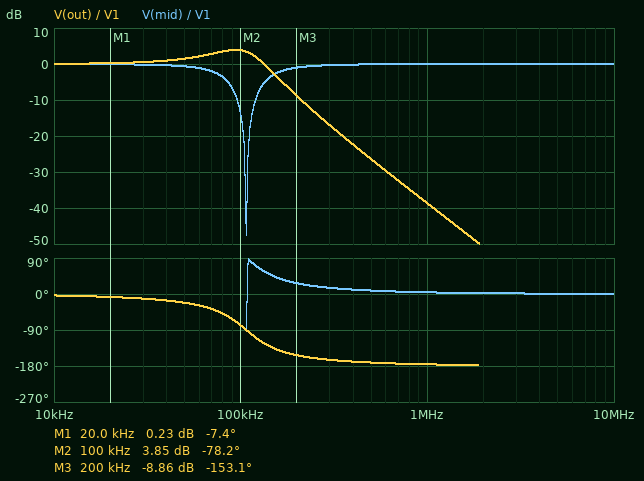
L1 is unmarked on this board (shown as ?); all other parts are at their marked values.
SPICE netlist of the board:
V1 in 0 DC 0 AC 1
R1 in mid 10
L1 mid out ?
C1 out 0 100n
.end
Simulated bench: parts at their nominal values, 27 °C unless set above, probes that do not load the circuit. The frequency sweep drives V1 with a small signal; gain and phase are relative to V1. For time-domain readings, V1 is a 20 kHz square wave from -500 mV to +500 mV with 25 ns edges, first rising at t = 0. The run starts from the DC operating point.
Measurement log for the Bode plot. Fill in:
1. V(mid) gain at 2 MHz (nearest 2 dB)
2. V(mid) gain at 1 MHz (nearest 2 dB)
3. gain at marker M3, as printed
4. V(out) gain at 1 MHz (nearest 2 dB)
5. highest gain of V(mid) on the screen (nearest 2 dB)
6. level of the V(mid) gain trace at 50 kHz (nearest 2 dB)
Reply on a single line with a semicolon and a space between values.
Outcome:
0 dB; 0 dB; -8.86 dB; -38 dB; 0 dB; 0 dB
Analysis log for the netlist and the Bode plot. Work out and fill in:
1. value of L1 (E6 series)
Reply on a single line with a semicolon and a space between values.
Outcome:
22 µH
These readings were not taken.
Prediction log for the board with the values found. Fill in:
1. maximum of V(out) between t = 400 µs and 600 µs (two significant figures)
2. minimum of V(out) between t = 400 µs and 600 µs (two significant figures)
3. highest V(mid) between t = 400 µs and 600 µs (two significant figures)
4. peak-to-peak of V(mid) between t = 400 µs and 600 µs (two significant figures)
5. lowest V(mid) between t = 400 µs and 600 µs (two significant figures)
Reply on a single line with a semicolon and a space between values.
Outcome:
830 mV; -830 mV; 640 mV; 1.3 V; -640 mV
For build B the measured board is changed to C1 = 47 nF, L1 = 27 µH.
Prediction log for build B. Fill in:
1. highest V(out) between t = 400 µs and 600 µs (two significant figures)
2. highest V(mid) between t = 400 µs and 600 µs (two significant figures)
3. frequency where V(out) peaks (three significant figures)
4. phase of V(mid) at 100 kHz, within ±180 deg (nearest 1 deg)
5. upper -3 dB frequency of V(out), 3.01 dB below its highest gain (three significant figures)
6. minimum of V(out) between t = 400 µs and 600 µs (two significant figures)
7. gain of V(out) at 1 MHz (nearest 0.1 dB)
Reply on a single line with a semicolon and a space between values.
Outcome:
1.0 V; 660 mV; 135 kHz; -31 deg; 162 kHz; -1.0 V; -33.8 dB
